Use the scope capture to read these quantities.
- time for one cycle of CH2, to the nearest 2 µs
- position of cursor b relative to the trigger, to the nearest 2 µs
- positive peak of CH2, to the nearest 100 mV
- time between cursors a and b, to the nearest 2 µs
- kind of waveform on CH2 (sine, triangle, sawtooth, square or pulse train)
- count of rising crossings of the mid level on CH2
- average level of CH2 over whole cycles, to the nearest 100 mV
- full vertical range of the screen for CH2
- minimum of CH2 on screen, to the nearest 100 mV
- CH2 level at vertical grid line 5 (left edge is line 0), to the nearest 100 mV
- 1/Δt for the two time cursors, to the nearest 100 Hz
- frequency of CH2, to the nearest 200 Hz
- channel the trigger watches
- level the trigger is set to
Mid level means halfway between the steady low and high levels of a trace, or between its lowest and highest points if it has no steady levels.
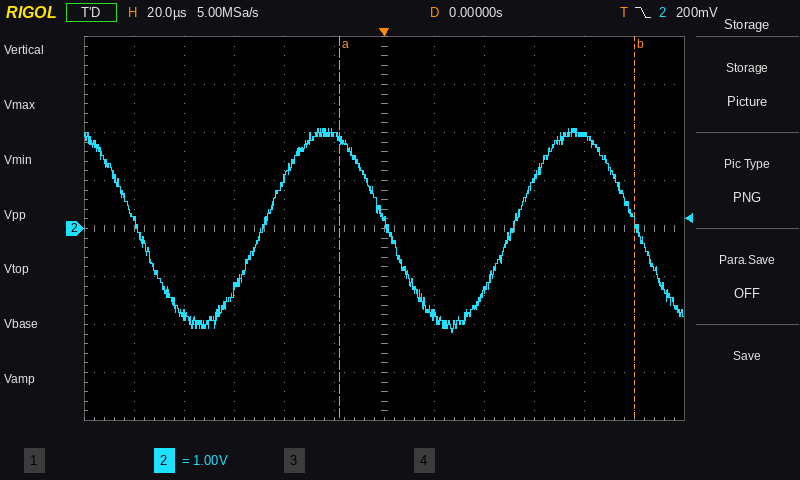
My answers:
100 µs
+100 µs
2.1 V
118 µs
sine
2
0.0 V
8 V
-2.2 V
2.0 V
8.5 kHz
10.0 kHz
CH2
200 mV
